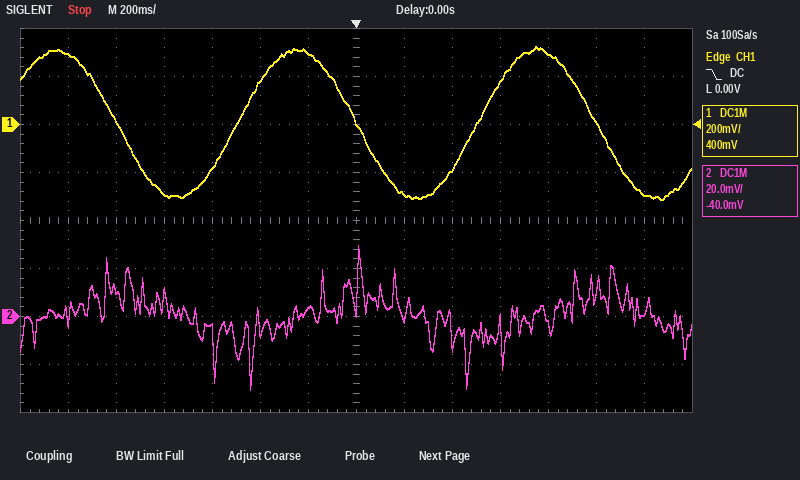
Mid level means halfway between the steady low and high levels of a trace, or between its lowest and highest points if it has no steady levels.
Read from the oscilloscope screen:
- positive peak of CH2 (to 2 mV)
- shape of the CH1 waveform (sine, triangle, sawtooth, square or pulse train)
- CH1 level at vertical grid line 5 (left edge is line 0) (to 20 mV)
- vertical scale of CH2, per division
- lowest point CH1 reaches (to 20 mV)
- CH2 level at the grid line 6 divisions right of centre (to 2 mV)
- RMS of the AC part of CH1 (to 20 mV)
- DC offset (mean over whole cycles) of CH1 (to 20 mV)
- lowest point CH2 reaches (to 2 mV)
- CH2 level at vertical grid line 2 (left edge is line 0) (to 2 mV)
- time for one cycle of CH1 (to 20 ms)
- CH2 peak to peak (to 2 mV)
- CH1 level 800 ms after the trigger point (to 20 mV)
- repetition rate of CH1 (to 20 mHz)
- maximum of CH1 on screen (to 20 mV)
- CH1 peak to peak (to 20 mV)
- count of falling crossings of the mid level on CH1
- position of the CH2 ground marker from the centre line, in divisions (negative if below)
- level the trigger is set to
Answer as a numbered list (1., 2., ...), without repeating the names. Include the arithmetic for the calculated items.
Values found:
1. 30 mV
2. sine
3. 180 mV
4. 20 mV
5. -320 mV
6. 2 mV
7. 640 mV / (2√2) ≈ 226 mV, so 220 mV to the nearest 20 mV
8. (320 mV + (-320 mV)) / 2 ≈ 0 mV
9. -30 mV
10. 12 mV
11. 1.00 s
12. 30 mV − (-30 mV) = 60 mV
13. 300 mV
14. 1 / 1.00 s ≈ 1.00 Hz
15. 320 mV
16. 320 mV − (-320 mV) = 640 mV
17. 3
18. -2.0 div
19. 0.00 V
